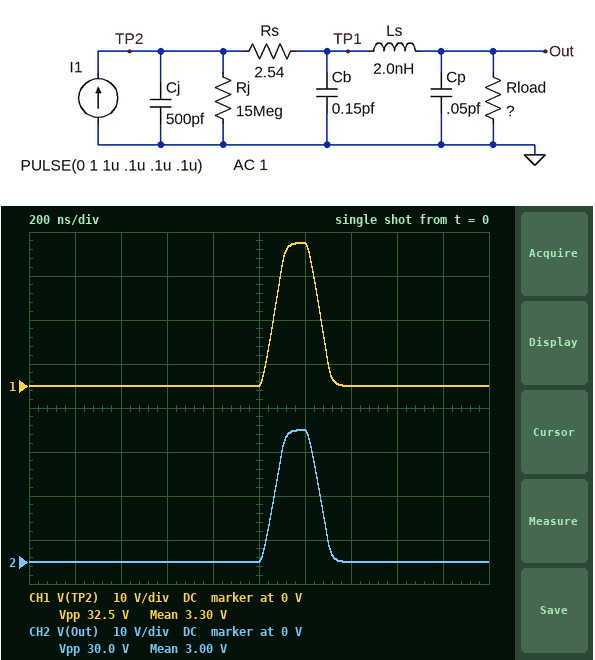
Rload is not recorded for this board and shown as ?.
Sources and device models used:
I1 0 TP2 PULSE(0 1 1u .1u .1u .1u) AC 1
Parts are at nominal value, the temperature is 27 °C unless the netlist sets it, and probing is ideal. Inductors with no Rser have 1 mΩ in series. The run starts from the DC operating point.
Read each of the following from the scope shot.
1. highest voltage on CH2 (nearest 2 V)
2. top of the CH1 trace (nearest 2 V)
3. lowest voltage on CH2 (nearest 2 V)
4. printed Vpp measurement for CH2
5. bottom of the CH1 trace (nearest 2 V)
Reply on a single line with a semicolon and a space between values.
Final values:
30 V; 32 V; 0 V; 30.0 V; 0 V
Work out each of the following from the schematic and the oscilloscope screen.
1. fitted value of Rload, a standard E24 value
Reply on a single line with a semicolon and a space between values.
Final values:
30 Ω
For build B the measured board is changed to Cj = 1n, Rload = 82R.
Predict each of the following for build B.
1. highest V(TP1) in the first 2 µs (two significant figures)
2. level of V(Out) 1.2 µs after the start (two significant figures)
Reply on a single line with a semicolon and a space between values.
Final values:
69 V; 67 V
